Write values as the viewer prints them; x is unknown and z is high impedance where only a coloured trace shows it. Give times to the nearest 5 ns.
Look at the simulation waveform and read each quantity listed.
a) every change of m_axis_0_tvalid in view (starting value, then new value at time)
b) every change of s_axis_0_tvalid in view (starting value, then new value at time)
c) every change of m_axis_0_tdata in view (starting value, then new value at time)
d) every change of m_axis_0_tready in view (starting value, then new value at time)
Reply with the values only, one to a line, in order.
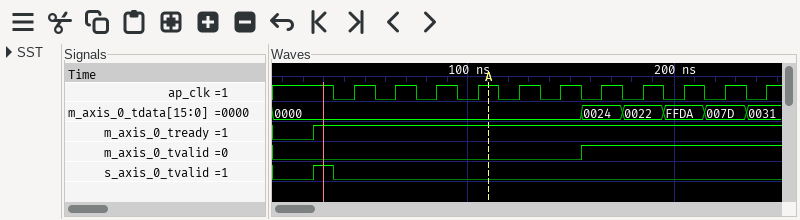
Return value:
0, 1 at 155 ns
0, 1 at 25 ns, 0 at 35 ns
0000, 0024 at 155 ns, 0022 at 175 ns, FFDA at 195 ns, 007D at 215 ns, 0031 at 235 ns
0, 1 at 25 ns
